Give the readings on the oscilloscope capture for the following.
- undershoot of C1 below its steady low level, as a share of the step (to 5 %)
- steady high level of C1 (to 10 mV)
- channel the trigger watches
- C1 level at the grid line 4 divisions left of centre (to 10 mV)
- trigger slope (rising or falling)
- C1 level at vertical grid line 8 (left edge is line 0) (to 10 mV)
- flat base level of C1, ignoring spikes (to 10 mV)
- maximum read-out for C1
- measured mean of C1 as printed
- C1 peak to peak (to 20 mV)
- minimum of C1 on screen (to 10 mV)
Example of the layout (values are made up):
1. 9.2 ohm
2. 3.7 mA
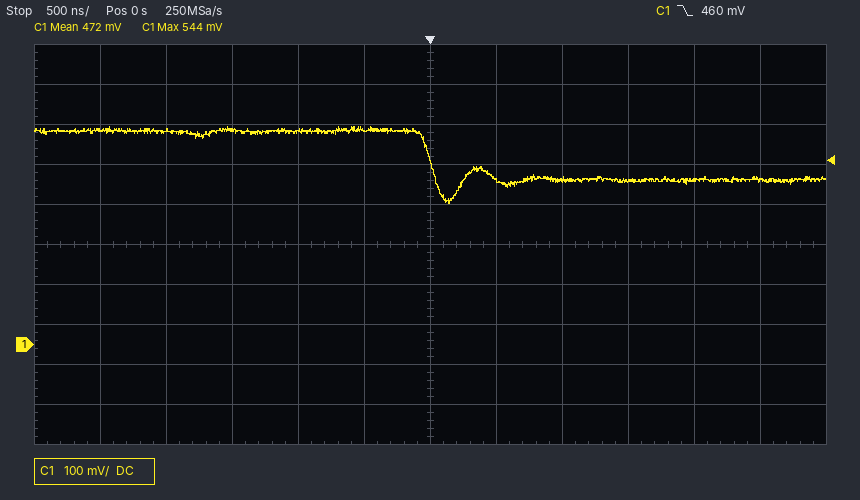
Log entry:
1. 50 %
2. 530 mV
3. C1
4. 530 mV
5. falling
6. 410 mV
7. 410 mV
8. 544 mV
9. 472 mV
10. 200 mV
11. 350 mV
